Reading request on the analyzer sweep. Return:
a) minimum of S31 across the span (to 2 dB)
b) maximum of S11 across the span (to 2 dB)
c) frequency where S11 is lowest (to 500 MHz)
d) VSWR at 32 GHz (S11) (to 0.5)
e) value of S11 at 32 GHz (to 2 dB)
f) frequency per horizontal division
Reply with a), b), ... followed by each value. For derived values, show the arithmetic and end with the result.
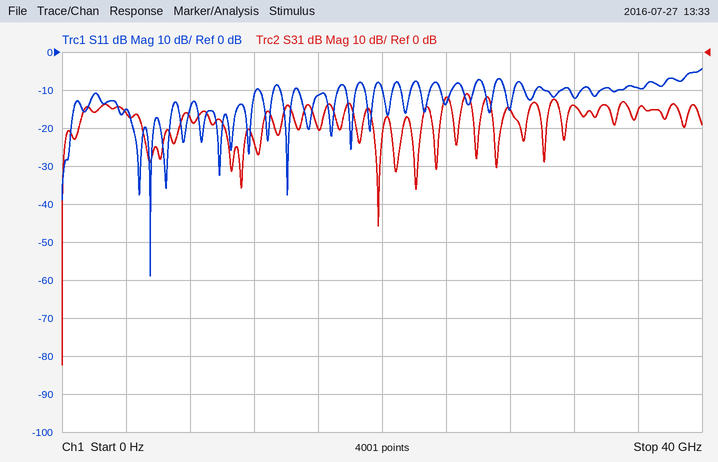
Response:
a) -82 dB
b) -4 dB
c) 5.5 GHz
d) |Γ| = 10^(-12/20) = 0.2512; VSWR = (1 + 0.2512)/(1 − 0.2512) ≈ 1.67, so 1.5 to the nearest 0.5
e) -12 dB
f) 4 GHz
